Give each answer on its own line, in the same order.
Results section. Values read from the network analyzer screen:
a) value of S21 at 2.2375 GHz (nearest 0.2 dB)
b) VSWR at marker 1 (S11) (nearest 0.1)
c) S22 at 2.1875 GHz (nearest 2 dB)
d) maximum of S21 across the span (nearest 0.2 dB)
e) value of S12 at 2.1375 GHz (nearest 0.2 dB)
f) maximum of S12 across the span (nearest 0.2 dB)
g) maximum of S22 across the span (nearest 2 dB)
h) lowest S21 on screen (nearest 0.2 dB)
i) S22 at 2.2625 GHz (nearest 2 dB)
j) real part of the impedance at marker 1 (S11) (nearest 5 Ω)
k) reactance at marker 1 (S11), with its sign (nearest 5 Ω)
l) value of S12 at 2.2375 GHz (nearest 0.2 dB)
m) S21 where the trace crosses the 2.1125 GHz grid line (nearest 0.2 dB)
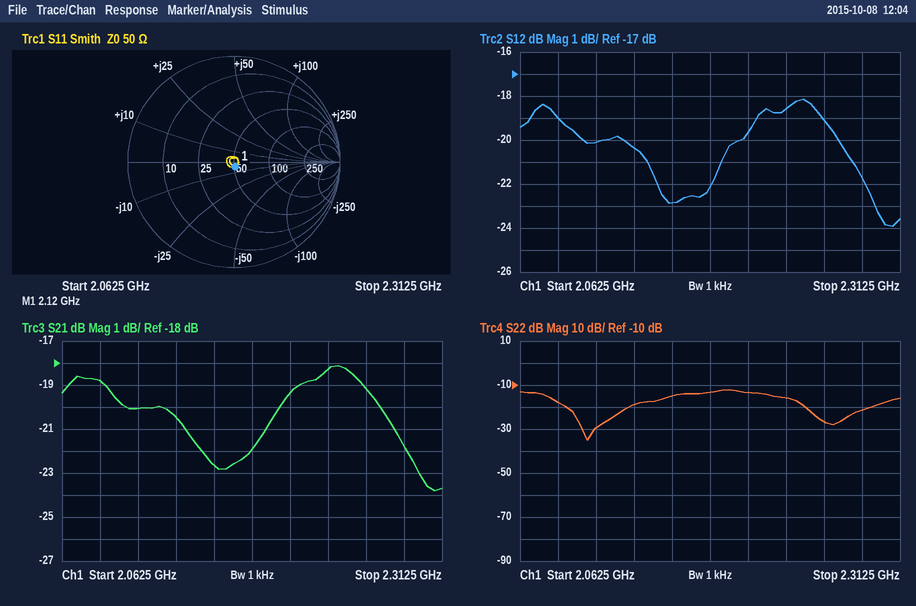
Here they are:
-18.2 dB
1.1
-14 dB
-18.2 dB
-20.4 dB
-18.2 dB
-12 dB
-23.8 dB
-26 dB
50 Ω
-5 Ω
-18.6 dB
-20.0 dB
